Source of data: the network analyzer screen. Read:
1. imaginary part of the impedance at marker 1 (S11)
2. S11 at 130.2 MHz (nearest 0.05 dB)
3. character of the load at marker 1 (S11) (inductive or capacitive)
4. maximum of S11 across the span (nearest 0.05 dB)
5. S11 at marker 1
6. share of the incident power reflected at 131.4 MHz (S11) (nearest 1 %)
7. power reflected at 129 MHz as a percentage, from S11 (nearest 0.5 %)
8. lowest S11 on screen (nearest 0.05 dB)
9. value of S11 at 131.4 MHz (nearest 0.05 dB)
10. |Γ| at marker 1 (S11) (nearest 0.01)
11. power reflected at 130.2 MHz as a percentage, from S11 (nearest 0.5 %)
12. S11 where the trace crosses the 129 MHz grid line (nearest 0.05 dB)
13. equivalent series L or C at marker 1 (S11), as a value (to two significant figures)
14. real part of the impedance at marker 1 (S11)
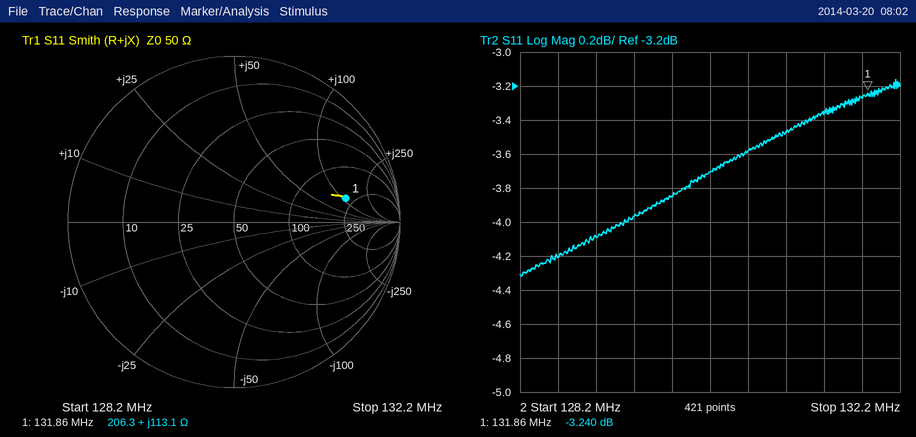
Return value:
+113.1 Ω
-3.70 dB
inductive
-3.15 dB
-3.240 dB
46 %
39.0 %
-4.30 dB
-3.35 dB
0.69
42.5 %
-4.10 dB
140 nH
206.3 Ω
